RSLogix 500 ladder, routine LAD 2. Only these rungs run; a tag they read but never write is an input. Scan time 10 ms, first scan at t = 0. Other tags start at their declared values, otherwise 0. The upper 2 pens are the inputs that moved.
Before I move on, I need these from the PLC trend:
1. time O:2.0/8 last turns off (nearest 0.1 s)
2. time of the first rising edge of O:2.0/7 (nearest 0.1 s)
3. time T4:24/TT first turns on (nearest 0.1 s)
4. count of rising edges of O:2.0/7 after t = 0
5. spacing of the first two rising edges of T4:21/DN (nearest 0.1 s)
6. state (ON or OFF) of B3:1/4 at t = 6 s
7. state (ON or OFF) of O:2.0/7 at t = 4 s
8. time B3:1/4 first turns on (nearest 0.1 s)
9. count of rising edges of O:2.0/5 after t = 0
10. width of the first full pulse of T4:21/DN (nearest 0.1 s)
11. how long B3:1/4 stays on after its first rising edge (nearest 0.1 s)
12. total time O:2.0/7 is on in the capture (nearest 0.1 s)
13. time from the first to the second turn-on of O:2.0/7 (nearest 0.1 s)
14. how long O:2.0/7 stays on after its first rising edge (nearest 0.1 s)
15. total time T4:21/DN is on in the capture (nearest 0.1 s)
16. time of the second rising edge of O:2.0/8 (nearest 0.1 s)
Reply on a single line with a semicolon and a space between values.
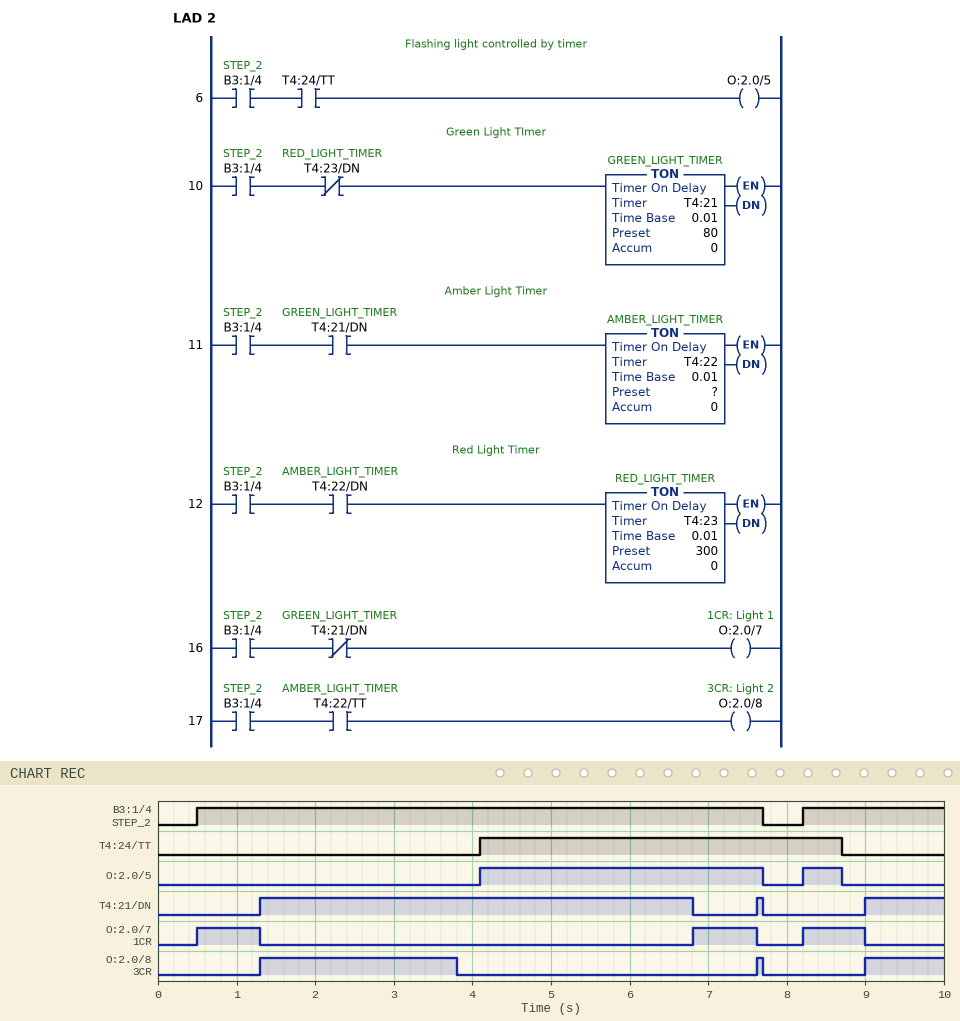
7.7 s; 0.5 s; 4.1 s; 3; 6.3 s; ON; OFF; 0.5 s; 2; 5.5 s; 7.2 s; 2.4 s; 6.3 s; 0.8 s; 6.6 s; 7.6 s
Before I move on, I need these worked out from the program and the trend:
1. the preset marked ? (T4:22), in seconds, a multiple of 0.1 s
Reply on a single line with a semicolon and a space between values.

2.5 s
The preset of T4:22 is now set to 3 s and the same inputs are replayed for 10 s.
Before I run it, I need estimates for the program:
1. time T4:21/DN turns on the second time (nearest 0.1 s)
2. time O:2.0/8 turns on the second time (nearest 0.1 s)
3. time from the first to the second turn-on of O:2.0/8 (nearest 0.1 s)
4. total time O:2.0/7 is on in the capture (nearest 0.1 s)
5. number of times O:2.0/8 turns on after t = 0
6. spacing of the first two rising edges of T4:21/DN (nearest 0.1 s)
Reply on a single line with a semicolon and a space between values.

9.0 s; 9.0 s; 7.7 s; 2.0 s; 2; 7.7 s
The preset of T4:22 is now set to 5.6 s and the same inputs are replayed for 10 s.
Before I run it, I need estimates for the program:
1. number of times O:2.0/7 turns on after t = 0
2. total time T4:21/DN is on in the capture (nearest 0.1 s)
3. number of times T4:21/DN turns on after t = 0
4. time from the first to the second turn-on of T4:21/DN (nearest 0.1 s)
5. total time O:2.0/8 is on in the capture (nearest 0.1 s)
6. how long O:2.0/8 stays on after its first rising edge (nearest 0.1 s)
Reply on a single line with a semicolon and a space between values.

2; 7.4 s; 2; 7.7 s; 6.6 s; 5.6 s
